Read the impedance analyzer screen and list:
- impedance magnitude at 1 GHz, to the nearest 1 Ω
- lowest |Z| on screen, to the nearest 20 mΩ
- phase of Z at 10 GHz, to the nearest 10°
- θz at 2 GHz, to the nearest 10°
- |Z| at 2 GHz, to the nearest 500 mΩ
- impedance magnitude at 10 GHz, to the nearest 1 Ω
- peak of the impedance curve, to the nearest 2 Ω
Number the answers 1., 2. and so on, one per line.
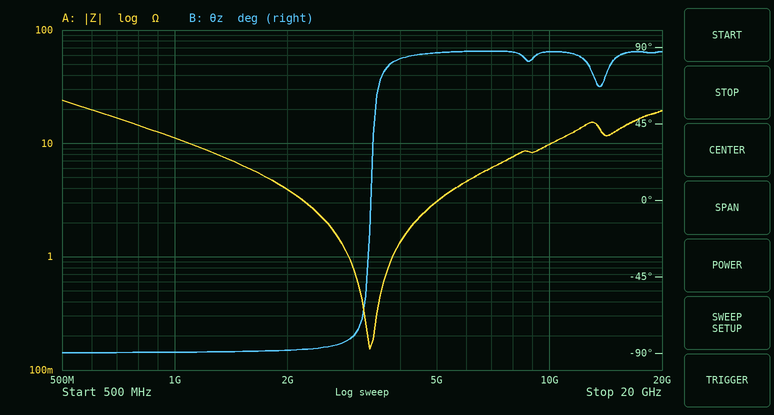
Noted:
1. 11 Ω
2. 160 mΩ
3. 90°
4. -90°
5. 4.0 Ω
6. 10 Ω
7. 24 Ω
